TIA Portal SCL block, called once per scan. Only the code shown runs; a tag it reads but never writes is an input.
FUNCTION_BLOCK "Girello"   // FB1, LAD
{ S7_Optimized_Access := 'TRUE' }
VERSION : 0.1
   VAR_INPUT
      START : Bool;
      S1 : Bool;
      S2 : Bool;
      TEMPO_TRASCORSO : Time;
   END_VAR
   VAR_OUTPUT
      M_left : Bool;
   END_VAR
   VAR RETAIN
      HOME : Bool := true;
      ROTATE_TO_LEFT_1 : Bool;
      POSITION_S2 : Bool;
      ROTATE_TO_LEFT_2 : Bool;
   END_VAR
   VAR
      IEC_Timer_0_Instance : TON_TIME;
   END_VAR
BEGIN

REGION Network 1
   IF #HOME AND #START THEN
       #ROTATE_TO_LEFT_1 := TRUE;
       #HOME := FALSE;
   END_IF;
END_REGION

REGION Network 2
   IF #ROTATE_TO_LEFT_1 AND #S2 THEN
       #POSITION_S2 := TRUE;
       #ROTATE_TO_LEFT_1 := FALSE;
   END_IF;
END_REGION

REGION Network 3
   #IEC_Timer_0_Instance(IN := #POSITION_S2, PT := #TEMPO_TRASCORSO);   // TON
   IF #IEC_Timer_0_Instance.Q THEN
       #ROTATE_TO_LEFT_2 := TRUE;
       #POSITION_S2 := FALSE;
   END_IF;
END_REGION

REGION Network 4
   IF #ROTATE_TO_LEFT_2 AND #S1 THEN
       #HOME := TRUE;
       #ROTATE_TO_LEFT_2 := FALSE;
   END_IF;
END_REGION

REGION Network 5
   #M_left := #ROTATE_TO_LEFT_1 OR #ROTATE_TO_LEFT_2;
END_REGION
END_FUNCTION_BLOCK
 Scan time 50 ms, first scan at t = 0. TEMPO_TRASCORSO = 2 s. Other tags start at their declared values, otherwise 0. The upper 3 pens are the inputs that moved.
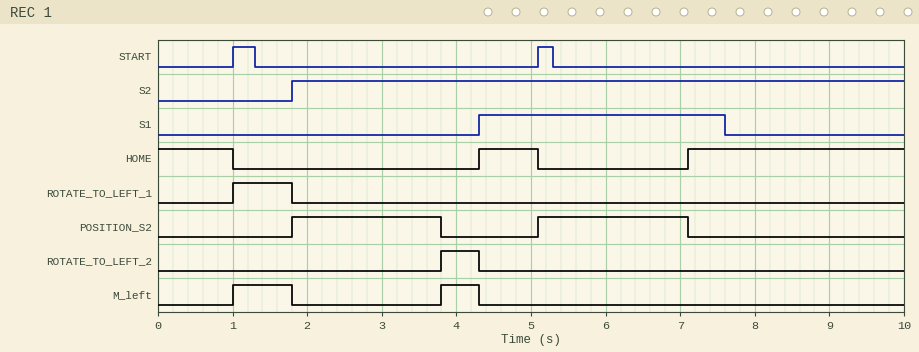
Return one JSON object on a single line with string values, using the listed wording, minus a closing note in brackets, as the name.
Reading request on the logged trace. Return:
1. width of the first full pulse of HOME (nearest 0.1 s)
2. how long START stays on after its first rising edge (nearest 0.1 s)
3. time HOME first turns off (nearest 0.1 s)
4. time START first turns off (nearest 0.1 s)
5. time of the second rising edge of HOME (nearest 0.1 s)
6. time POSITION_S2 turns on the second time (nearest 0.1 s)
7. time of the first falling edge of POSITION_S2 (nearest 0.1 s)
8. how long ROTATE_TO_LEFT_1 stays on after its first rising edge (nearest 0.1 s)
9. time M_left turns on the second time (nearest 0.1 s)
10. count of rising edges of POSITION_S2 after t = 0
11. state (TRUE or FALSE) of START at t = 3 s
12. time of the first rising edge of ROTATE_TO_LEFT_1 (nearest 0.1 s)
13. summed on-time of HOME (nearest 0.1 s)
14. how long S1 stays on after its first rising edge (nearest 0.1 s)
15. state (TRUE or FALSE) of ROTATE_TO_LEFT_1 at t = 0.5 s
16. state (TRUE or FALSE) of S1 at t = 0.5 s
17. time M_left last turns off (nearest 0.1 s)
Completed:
{"width of the first full pulse of HOME": "0.8 s", "how long START stays on after its first rising edge": "0.3 s", "time HOME first turns off": "1.0 s", "time START first turns off": "1.3 s", "time of the second rising edge of HOME": "7.1 s", "time POSITION_S2 turns on the second time": "5.1 s", "time of the first falling edge of POSITION_S2": "3.8 s", "how long ROTATE_TO_LEFT_1 stays on after its first rising edge": "0.8 s", "time M_left turns on the second time": "3.8 s", "count of rising edges of POSITION_S2 after t = 0": "2", "state (TRUE or FALSE) of START at t = 3 s": "FALSE", "time of the first rising edge of ROTATE_TO_LEFT_1": "1.0 s", "summed on-time of HOME": "4.7 s", "how long S1 stays on after its first rising edge": "3.3 s", "state (TRUE or FALSE) of ROTATE_TO_LEFT_1 at t = 0.5 s": "FALSE", "state (TRUE or FALSE) of S1 at t = 0.5 s": "FALSE", "time M_left last turns off": "4.3 s"}
